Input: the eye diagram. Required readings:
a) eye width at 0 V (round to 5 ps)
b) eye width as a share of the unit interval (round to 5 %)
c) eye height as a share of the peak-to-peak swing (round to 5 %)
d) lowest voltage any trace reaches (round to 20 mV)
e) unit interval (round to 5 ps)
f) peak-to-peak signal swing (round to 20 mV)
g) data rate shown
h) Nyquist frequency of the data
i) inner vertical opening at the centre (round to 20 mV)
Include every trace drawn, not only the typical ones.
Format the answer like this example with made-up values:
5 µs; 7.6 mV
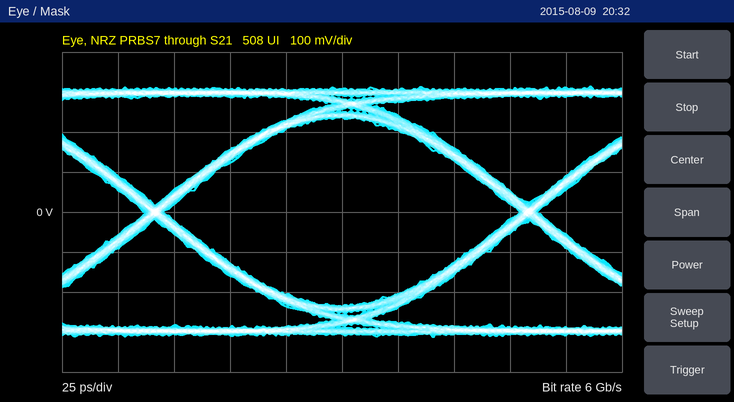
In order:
160 ps; 95 %; 75 %; -320 mV; 165 ps; 620 mV; 6 Gb/s; 3 GHz; 480 mV
